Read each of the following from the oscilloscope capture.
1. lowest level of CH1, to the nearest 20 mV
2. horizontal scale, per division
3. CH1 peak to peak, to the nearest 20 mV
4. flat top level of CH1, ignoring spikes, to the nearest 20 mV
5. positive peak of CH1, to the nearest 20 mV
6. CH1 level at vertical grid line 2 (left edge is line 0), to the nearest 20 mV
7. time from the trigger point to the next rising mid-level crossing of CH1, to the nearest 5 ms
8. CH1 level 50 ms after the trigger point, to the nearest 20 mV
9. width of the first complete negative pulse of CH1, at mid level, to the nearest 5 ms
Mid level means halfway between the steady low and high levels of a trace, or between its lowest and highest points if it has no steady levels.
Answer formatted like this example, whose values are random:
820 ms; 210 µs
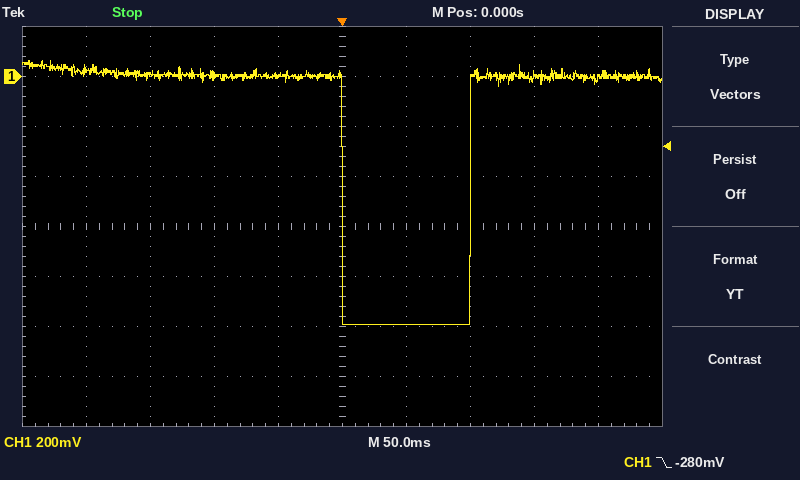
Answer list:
-1.00 V; 50 ms; 1.06 V; 0 mV; 60 mV; 0 mV; 100 ms; -1.00 V; 100 ms
